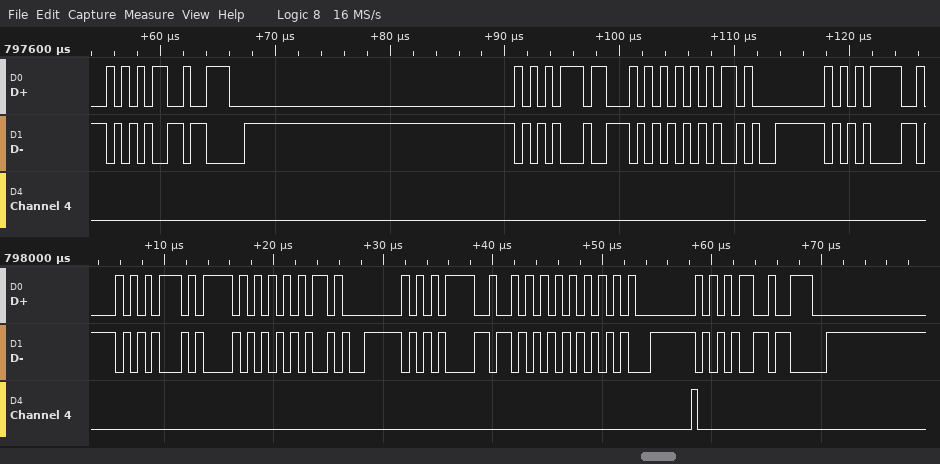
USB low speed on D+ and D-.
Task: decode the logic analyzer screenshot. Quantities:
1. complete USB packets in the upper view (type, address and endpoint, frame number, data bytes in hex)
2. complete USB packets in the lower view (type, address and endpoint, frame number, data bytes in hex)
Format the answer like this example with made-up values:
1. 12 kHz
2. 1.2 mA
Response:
1. ACK, IN ADDR 0 EP 0
2. OUT ADDR 0 EP 0, DATA1 [ ], ACK
